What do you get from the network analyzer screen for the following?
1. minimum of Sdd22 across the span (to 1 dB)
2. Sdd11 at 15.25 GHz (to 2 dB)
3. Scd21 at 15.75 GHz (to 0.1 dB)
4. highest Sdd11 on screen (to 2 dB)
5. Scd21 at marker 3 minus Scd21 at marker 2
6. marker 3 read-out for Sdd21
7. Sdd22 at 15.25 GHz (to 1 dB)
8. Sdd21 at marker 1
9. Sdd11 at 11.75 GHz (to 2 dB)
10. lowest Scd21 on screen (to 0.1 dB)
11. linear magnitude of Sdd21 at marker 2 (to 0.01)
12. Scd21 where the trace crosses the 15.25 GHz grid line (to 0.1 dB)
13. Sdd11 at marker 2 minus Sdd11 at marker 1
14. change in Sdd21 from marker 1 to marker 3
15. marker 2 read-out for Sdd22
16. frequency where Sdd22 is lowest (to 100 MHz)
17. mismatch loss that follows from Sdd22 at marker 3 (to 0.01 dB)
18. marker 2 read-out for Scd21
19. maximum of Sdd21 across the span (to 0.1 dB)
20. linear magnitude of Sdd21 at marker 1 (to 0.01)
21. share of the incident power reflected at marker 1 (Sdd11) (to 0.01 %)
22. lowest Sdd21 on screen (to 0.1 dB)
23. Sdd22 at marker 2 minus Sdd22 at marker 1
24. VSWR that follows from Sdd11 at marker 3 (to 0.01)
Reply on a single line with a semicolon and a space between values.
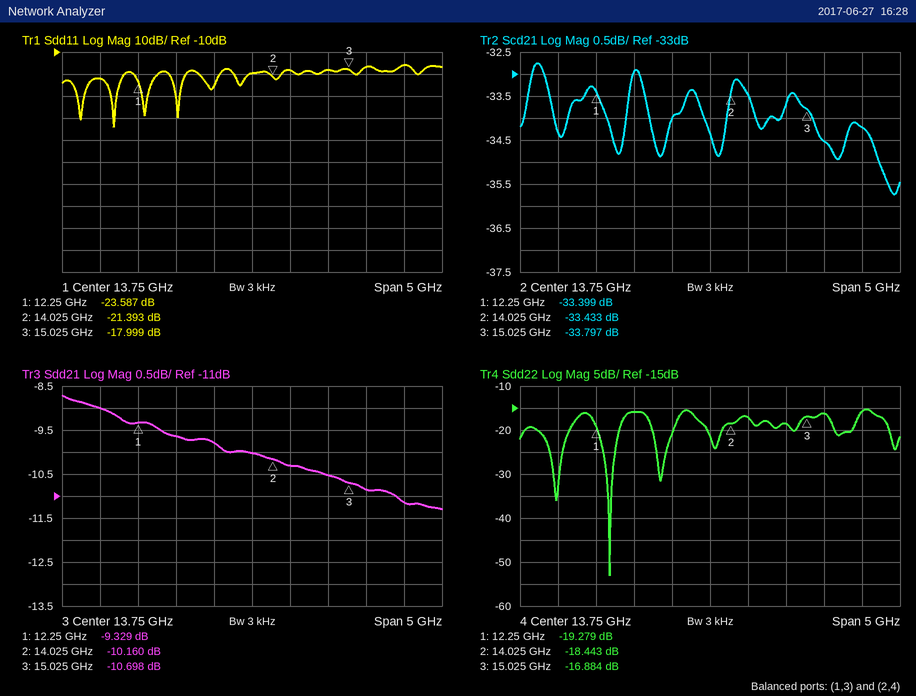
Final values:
-53 dB; -16 dB; -34.2 dB; -16 dB; -0.364 dB; -10.698 dB; -16 dB; -9.329 dB; -22 dB; -35.7 dB; 0.31; -34.5 dB; 2.194 dB; -1.369 dB; -18.443 dB; 12.4 GHz; 0.09 dB; -33.433 dB; -8.7 dB; 0.34; 0.44 %; -11.3 dB; 0.836 dB; 1.29
